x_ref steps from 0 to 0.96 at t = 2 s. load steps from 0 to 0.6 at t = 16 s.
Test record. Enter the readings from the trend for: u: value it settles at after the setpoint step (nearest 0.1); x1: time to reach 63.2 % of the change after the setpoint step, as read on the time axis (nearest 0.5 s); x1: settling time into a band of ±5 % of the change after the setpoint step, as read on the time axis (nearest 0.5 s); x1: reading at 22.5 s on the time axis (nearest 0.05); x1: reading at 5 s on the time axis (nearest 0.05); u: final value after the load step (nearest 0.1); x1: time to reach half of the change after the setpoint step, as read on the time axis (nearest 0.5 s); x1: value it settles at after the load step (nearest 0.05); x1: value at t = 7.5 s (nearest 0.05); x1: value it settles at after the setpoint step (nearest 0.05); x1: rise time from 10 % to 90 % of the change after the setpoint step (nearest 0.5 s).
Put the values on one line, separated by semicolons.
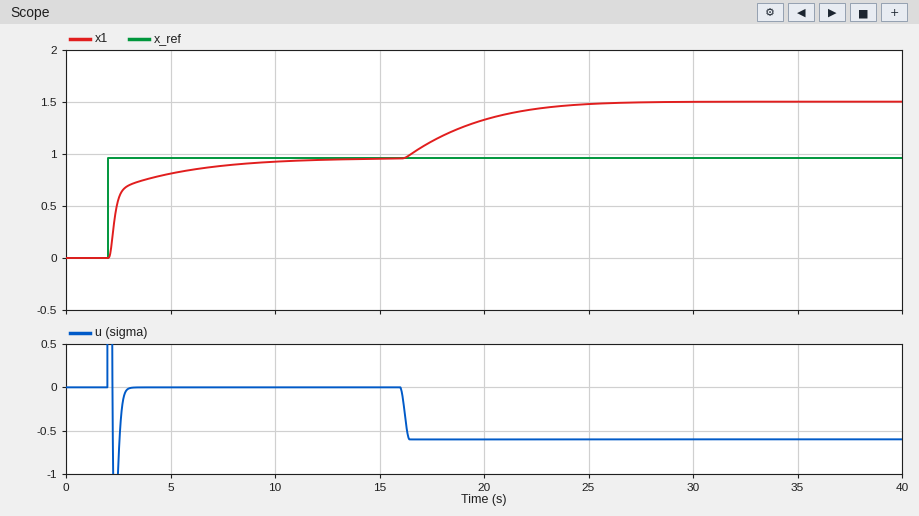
0.0; 2.5 s; 9.0 s; 1.45; 0.80; -0.6; 2.5 s; 1.50; 0.90; 0.95; 4.5 s
